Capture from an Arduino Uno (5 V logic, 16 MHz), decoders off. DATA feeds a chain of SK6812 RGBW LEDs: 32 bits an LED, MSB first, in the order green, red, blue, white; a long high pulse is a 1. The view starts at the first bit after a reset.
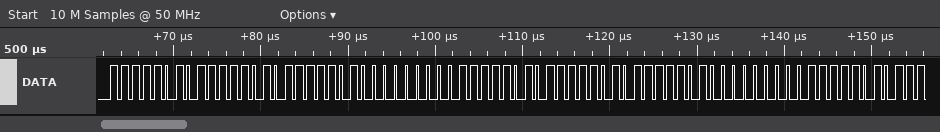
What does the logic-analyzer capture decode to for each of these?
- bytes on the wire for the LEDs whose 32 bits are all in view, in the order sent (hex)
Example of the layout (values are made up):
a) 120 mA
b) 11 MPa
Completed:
a) FA FA FA 00 FA FA FA 00
